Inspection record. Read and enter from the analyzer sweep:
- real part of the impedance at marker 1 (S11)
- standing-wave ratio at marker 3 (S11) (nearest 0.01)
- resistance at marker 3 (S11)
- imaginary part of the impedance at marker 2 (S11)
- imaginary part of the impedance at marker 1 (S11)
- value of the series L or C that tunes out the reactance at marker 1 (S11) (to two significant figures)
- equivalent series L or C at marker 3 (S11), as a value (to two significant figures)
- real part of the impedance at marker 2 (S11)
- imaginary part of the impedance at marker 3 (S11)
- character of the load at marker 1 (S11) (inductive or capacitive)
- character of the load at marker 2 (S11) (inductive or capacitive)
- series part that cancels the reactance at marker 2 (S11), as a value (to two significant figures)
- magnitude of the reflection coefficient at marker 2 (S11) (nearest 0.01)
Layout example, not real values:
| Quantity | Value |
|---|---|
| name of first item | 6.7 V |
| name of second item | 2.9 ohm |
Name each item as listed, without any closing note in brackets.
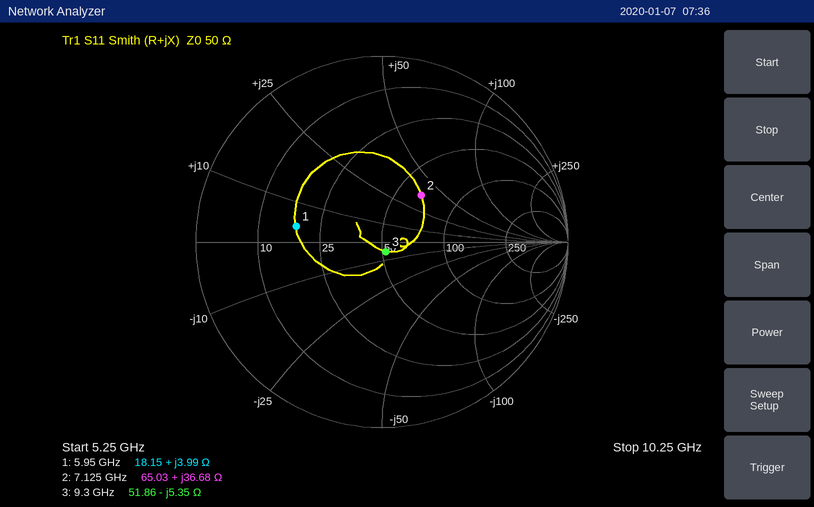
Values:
| Quantity | Value |
|---|---|
| real part of the impedance at marker 1 | 18.15 Ω |
| standing-wave ratio at marker 3 (S11) | 1.12 |
| resistance at marker 3 | 51.86 Ω |
| imaginary part of the impedance at marker 2 | +36.68 Ω |
| imaginary part of the impedance at marker 1 | +3.99 Ω |
| value of the series L or C that tunes out the reactance at marker 1 (S11) | 6.7 pF |
| equivalent series L or C at marker 3 (S11), as a value | 3.2 pF |
| real part of the impedance at marker 2 | 65.03 Ω |
| imaginary part of the impedance at marker 3 | -5.35 Ω |
| character of the load at marker 1 (S11) | inductive |
| character of the load at marker 2 (S11) | inductive |
| series part that cancels the reactance at marker 2 (S11), as a value | 610 fF |
| magnitude of the reflection coefficient at marker 2 (S11) | 0.33 |
